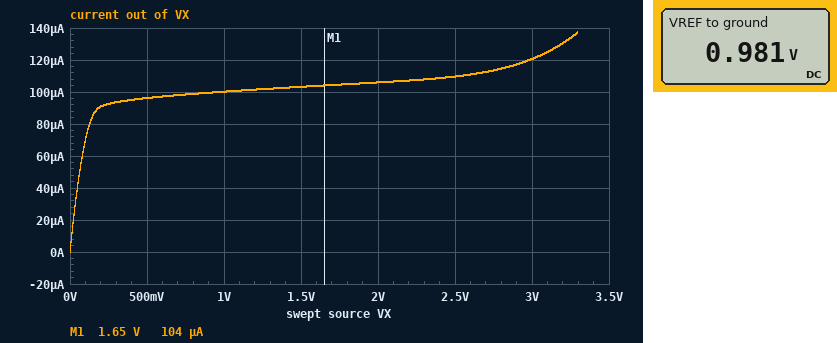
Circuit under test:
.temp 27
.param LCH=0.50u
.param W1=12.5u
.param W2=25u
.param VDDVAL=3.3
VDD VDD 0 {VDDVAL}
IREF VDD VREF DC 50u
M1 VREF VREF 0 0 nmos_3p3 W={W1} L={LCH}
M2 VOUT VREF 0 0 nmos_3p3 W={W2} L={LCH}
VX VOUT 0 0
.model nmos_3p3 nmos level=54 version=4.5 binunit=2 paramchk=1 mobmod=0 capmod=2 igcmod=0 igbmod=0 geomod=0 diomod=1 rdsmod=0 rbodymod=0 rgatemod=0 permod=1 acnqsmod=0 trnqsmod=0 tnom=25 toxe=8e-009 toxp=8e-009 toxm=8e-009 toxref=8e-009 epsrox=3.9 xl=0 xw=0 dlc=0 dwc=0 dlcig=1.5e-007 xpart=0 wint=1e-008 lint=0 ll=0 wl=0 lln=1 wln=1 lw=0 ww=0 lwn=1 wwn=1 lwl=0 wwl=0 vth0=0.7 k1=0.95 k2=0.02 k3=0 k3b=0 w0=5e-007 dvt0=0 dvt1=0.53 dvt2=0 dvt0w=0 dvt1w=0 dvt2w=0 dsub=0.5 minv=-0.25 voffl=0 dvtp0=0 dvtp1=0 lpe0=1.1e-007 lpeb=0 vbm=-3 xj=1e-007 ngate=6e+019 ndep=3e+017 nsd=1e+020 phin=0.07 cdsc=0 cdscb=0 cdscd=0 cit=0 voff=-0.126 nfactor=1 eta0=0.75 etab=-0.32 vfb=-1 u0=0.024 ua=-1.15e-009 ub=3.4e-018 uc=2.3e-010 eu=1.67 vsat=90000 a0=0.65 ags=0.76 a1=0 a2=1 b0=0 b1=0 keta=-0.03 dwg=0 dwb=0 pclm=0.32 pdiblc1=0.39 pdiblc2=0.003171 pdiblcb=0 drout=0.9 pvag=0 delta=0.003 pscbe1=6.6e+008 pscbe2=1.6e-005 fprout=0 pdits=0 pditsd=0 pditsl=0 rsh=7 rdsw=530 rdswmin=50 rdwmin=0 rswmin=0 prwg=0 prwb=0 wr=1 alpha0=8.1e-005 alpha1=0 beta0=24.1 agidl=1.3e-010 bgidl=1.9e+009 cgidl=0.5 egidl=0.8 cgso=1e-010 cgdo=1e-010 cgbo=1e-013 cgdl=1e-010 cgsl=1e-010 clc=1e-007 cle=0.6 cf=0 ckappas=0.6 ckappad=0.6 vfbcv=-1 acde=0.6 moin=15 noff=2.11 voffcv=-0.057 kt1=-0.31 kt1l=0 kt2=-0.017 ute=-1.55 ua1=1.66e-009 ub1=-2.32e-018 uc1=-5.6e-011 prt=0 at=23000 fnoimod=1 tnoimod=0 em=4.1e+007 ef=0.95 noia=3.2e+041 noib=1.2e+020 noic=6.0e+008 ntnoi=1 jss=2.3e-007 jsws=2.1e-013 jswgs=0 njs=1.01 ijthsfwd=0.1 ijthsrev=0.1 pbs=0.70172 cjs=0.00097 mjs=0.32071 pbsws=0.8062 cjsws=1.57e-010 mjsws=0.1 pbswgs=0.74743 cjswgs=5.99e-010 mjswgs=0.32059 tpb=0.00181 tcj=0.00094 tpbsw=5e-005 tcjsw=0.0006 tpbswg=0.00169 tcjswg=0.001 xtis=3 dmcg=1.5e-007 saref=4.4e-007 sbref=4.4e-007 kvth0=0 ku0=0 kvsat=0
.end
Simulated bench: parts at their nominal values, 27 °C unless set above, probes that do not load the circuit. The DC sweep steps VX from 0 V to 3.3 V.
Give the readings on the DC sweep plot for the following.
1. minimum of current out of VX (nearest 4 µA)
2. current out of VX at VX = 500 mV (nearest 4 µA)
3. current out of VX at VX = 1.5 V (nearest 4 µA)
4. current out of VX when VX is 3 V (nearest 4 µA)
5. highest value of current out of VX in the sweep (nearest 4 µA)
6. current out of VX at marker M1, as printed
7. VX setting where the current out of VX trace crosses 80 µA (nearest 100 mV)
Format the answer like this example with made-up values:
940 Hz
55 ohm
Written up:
0 A
96 µA
104 µA
120 µA
136 µA
104 µA
100 mV
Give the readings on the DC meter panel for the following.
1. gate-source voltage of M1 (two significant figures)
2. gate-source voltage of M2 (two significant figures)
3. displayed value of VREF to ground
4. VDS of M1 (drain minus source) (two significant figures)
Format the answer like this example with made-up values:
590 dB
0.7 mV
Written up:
980 mV
980 mV
0.981 V
980 mV
